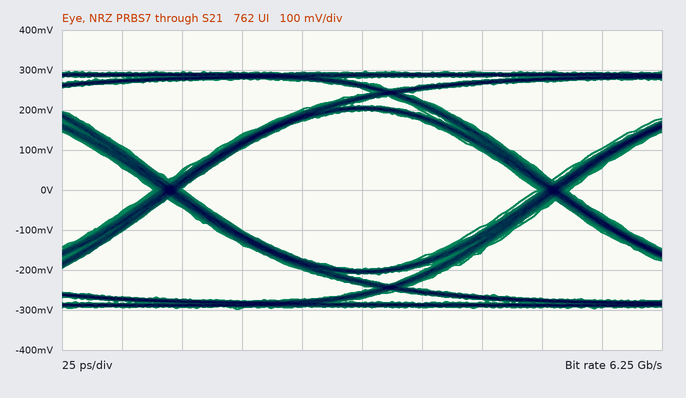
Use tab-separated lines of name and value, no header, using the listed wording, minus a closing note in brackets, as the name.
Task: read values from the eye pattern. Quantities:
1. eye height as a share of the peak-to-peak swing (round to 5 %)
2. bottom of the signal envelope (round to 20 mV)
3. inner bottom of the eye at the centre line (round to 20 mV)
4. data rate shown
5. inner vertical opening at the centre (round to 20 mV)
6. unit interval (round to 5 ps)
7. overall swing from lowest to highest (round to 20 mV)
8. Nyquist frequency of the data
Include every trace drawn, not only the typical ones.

eye height as a share of the peak-to-peak swing	65 %
bottom of the signal envelope	-300 mV
inner bottom of the eye at the centre line	-200 mV
data rate shown	6.25 Gb/s
inner vertical opening at the centre	400 mV
unit interval	160 ps
overall swing from lowest to highest	600 mV
Nyquist frequency of the data	3.125 GHz
